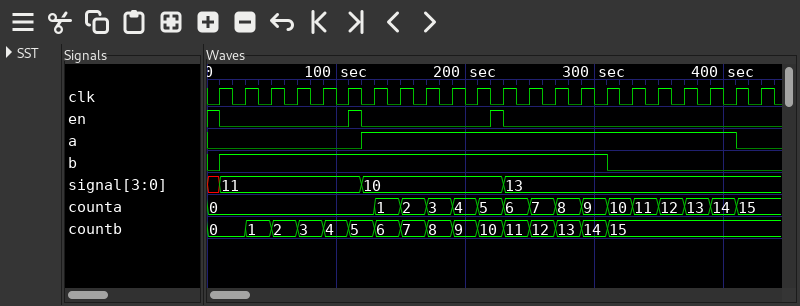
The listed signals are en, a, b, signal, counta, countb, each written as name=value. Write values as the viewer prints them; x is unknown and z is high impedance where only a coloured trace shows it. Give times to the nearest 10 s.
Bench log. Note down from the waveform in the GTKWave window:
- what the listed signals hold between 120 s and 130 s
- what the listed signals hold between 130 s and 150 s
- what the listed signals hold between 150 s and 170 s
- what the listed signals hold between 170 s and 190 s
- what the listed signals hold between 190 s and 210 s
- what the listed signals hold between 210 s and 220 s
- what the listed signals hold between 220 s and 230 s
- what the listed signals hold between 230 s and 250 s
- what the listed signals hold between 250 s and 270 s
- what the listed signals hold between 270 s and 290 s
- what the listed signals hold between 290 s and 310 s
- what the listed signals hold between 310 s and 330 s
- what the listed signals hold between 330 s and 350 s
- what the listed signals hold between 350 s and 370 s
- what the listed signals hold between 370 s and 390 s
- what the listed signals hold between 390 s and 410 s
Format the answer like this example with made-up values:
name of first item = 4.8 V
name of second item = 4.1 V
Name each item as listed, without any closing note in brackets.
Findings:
what the listed signals hold between 120 s and 130 s = en=0, a=1, b=1, signal=10, counta=0, countb=5
what the listed signals hold between 130 s and 150 s = en=0, a=1, b=1, signal=10, counta=1, countb=6
what the listed signals hold between 150 s and 170 s = en=0, a=1, b=1, signal=10, counta=2, countb=7
what the listed signals hold between 170 s and 190 s = en=0, a=1, b=1, signal=10, counta=3, countb=8
what the listed signals hold between 190 s and 210 s = en=0, a=1, b=1, signal=10, counta=4, countb=9
what the listed signals hold between 210 s and 220 s = en=0, a=1, b=1, signal=10, counta=5, countb=10
what the listed signals hold between 220 s and 230 s = en=1, a=1, b=1, signal=10, counta=5, countb=10
what the listed signals hold between 230 s and 250 s = en=0, a=1, b=1, signal=13, counta=6, countb=11
what the listed signals hold between 250 s and 270 s = en=0, a=1, b=1, signal=13, counta=7, countb=12
what the listed signals hold between 270 s and 290 s = en=0, a=1, b=1, signal=13, counta=8, countb=13
what the listed signals hold between 290 s and 310 s = en=0, a=1, b=1, signal=13, counta=9, countb=14
what the listed signals hold between 310 s and 330 s = en=0, a=1, b=0, signal=13, counta=10, countb=15
what the listed signals hold between 330 s and 350 s = en=0, a=1, b=0, signal=13, counta=11, countb=15
what the listed signals hold between 350 s and 370 s = en=0, a=1, b=0, signal=13, counta=12, countb=15
what the listed signals hold between 370 s and 390 s = en=0, a=1, b=0, signal=13, counta=13, countb=15
what the listed signals hold between 390 s and 410 s = en=0, a=1, b=0, signal=13, counta=14, countb=15
